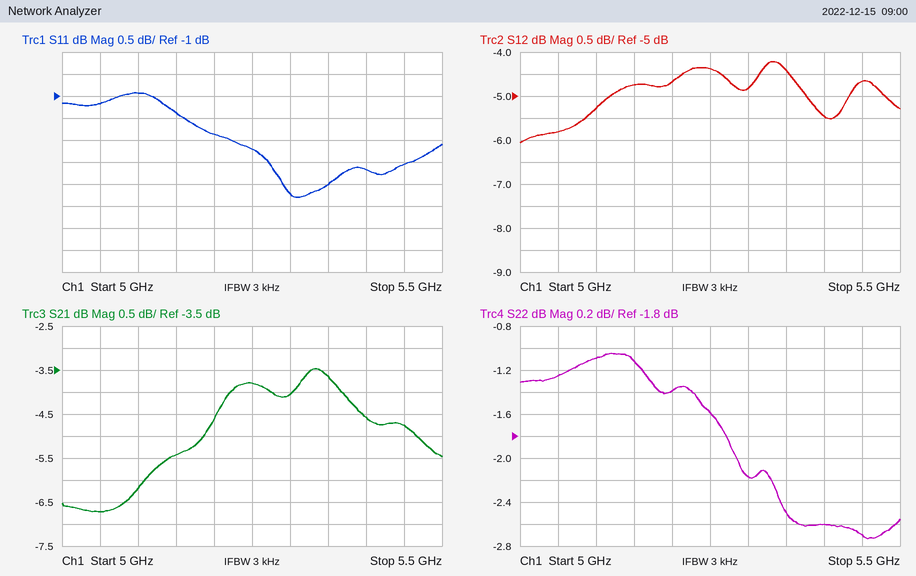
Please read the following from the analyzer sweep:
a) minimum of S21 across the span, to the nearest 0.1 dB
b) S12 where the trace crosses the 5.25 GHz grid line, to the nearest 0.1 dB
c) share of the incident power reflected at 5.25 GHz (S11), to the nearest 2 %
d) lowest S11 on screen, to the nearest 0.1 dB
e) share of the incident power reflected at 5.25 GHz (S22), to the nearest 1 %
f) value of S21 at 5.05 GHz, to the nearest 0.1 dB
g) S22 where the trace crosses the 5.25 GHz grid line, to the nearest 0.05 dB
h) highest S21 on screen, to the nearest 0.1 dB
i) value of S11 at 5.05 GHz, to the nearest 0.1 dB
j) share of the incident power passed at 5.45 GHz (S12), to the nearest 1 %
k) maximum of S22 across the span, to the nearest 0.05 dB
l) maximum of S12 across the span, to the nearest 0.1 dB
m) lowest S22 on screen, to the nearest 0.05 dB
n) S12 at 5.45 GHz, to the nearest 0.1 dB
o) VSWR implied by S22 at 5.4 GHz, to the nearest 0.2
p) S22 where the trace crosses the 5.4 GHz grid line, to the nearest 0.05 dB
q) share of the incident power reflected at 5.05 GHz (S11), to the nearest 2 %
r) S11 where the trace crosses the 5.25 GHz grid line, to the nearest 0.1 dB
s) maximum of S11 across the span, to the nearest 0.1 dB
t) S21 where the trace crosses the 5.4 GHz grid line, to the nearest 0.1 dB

-6.7 dB
-4.4 dB
60 %
-3.3 dB
69 %
-6.7 dB
-1.60 dB
-3.5 dB
-1.2 dB
34 %
-1.05 dB
-4.2 dB
-2.75 dB
-4.7 dB
6.8
-2.60 dB
76 %
-2.2 dB
-0.9 dB
-4.6 dB
